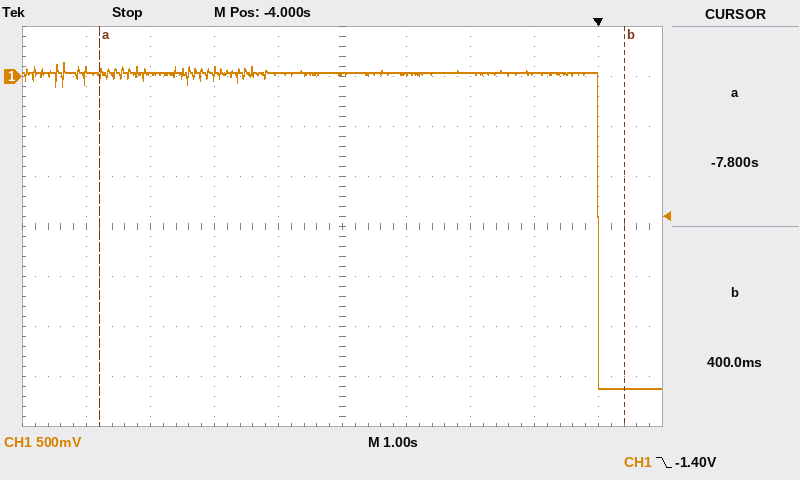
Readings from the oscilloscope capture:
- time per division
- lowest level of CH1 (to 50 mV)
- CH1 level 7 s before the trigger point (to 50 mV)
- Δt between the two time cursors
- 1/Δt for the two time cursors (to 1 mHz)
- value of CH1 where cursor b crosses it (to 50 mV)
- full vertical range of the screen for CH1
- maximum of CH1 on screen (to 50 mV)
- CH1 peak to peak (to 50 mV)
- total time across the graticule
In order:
1 s
-3.10 V
50 mV
8.2 s
122 mHz
-3.10 V
4 V
150 mV
3.25 V
10 s
